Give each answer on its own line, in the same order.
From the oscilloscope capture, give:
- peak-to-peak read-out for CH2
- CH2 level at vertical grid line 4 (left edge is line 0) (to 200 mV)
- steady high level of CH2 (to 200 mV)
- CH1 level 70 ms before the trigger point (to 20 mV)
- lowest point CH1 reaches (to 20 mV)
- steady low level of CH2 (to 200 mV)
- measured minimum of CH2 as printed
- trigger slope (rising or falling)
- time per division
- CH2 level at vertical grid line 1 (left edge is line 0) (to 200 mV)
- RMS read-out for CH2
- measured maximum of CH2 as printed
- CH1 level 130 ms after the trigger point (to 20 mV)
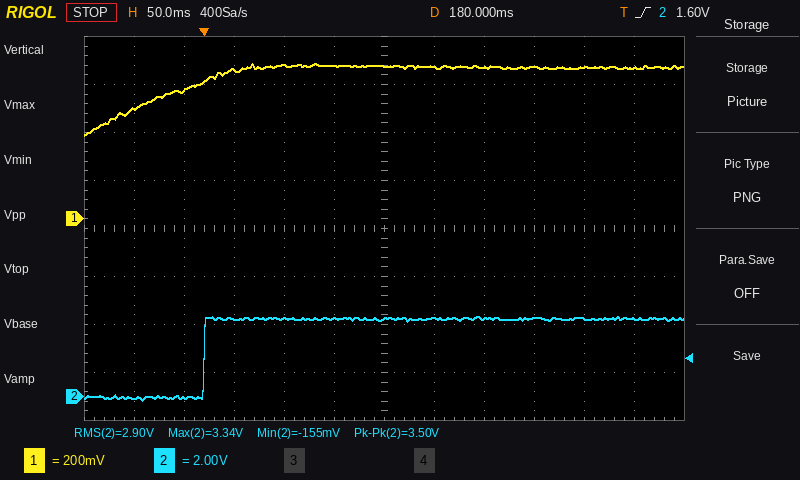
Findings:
3.50 V
3.2 V
3.2 V
460 mV
340 mV
0.0 V
-155 mV
rising
50 ms
0.0 V
2.90 V
3.34 V
640 mV
